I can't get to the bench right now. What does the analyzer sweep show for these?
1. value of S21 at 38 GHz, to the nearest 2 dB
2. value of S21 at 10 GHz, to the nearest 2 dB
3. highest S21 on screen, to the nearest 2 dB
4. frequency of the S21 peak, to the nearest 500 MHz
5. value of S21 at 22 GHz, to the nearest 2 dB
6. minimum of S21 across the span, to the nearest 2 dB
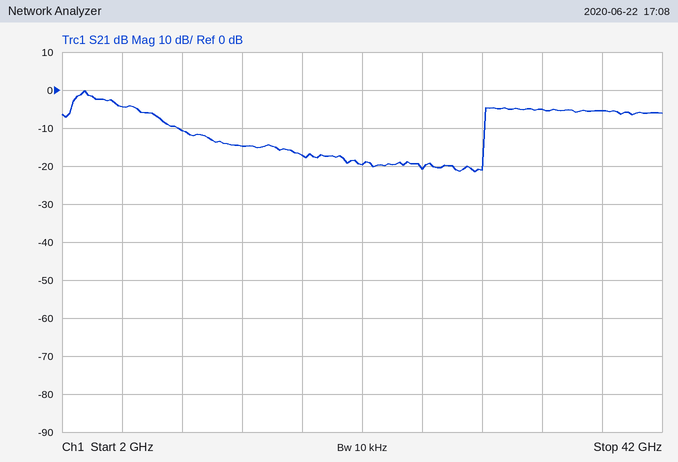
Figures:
-6 dB
-10 dB
0 dB
3.5 GHz
-20 dB
-22 dB
